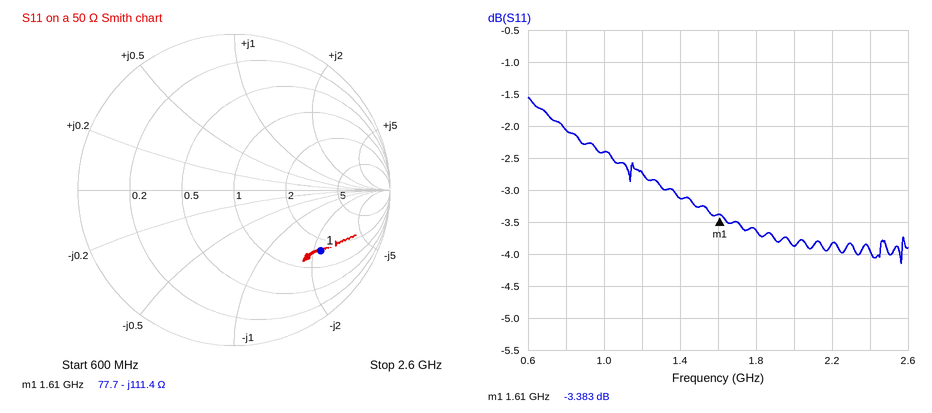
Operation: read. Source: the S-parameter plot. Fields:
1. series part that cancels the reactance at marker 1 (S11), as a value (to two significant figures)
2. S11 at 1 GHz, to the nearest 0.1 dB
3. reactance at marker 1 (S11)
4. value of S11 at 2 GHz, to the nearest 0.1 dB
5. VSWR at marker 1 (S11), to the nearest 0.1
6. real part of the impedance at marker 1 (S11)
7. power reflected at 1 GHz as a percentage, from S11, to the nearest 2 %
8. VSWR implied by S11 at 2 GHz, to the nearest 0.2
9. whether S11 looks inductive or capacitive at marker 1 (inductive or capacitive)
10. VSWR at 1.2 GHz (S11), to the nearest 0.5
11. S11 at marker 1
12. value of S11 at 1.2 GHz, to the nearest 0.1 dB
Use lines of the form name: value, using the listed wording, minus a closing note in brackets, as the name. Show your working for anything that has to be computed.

series part that cancels the reactance at marker 1 (S11), as a value: L = 111.4 Ω/(2π × 1.61 GHz) ≈ 11 nH
S11 at 1 GHz, to the nearest 0.1 dB: -2.4 dB
reactance at marker 1: -111.4 Ω
value of S11 at 2 GHz, to the nearest 0.1 dB: -3.9 dB
VSWR at marker 1 (S11), to the nearest 0.1: 5.2
real part of the impedance at marker 1: 77.7 Ω
power reflected at 1 GHz as a percentage, from S11, to the nearest 2 %: 10^(-2.4/10) ≈ 58 %
VSWR implied by S11 at 2 GHz, to the nearest 0.2: |Γ| = 10^(-3.9/20) = 0.6383; VSWR = (1 + 0.6383)/(1 − 0.6383) ≈ 4.53, so 4.6 to the nearest 0.2
whether S11 looks inductive or capacitive at marker 1: capacitive
VSWR at 1.2 GHz (S11), to the nearest 0.5: |Γ| = 10^(-2.7/20) = 0.7328; VSWR = (1 + 0.7328)/(1 − 0.7328) ≈ 6.5
S11 at marker 1: -3.383 dB
value of S11 at 1.2 GHz, to the nearest 0.1 dB: -2.7 dB
